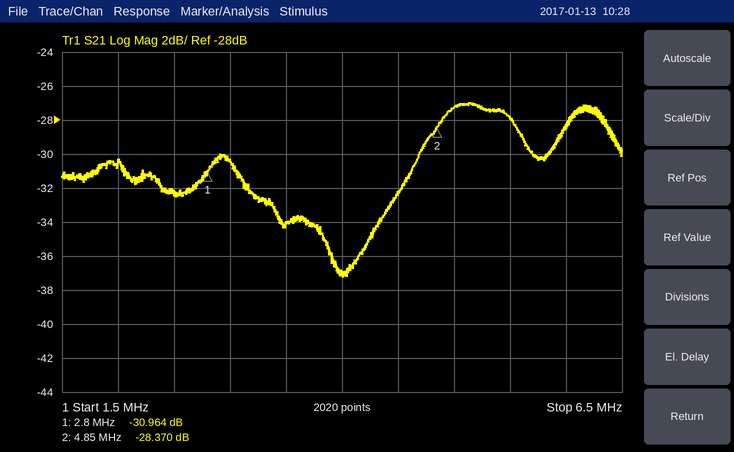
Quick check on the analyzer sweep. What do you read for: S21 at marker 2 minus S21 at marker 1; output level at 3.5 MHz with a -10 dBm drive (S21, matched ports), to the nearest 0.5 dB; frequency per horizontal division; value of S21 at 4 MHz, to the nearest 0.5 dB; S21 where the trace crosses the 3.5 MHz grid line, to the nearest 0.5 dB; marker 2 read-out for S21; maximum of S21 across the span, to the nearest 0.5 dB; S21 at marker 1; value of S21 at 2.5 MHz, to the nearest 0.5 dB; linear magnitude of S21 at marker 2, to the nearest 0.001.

2.594 dB
-44.0 dBm
500 kHz
-37.0 dB
-34.0 dB
-28.370 dB
-27.0 dB
-30.964 dB
-32.5 dB
0.038
